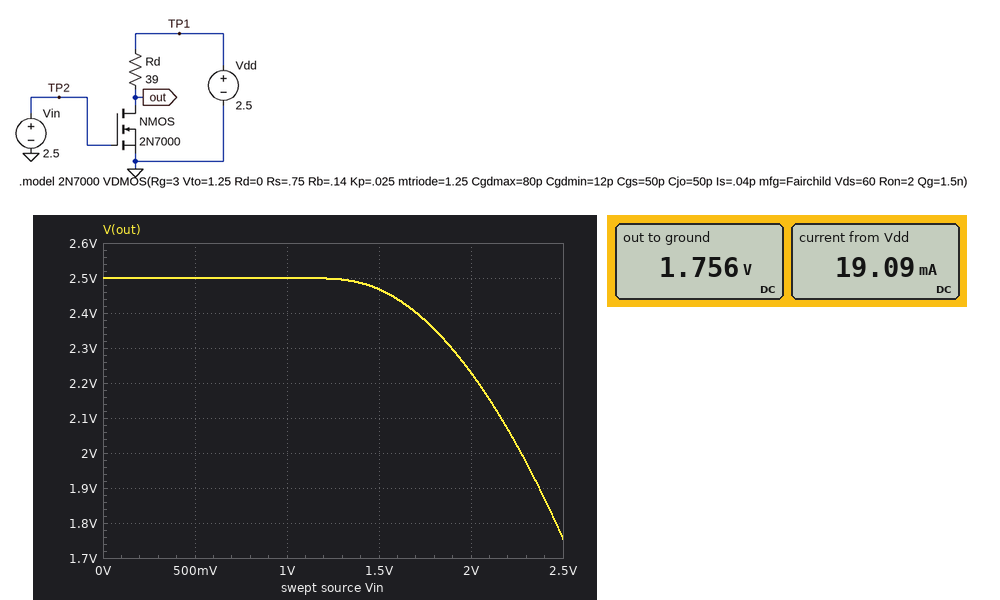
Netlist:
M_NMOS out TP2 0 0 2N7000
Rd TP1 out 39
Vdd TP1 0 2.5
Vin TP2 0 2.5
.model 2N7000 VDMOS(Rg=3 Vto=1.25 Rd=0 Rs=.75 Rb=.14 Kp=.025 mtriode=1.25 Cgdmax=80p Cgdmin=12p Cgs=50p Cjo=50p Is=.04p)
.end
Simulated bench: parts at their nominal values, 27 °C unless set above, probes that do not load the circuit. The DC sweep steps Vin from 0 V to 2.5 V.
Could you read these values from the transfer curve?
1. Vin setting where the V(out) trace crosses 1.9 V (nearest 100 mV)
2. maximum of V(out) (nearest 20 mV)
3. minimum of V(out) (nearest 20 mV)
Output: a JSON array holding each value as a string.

["2.4 V", "2.50 V", "1.76 V"]
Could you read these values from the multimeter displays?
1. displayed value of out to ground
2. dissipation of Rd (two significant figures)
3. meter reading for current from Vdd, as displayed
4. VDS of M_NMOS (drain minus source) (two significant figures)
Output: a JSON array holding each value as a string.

["1.756 V", "14 mW", "19.09 mA", "1.8 V"]
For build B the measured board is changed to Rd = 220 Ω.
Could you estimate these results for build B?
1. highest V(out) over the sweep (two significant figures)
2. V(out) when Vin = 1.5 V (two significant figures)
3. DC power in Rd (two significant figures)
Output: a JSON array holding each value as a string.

["2.5 V", "2.3 V", "22 mW"]
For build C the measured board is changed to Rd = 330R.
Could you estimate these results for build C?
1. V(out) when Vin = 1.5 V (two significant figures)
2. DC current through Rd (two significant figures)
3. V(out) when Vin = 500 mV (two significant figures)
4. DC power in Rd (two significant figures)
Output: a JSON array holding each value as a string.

["2.2 V", "7.0 mA", "2.5 V", "16 mW"]
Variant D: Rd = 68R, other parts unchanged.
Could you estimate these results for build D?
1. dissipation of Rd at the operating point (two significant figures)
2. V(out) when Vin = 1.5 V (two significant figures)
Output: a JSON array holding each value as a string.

["25 mW", "2.4 V"]
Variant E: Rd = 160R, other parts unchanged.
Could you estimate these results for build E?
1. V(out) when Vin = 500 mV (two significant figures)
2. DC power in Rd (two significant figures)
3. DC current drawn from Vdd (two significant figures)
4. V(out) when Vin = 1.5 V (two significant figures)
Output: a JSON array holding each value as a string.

["2.5 V", "27 mW", "13 mA", "2.4 V"]
